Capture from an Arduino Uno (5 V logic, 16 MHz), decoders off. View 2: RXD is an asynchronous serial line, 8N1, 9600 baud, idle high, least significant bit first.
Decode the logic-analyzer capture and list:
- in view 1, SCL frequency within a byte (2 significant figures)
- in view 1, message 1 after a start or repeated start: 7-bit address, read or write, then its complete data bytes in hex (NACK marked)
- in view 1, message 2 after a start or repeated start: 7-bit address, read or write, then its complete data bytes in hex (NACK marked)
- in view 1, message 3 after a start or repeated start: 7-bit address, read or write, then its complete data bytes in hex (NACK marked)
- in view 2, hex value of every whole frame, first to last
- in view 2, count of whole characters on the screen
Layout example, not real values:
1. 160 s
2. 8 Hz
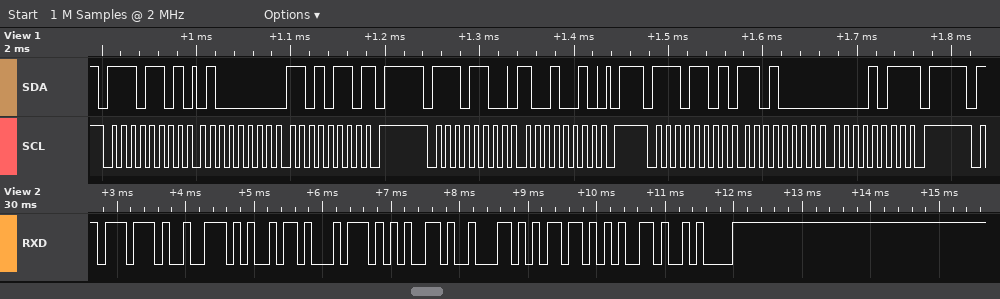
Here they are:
1. 100 kHz
2. 0x76 read: 40 D6 NACK
3. 0x76 write: 92
4. 0x76 read: D0 0B NACK
5. 77 72 69 74 65 62 6D 65 0A
6. 9
